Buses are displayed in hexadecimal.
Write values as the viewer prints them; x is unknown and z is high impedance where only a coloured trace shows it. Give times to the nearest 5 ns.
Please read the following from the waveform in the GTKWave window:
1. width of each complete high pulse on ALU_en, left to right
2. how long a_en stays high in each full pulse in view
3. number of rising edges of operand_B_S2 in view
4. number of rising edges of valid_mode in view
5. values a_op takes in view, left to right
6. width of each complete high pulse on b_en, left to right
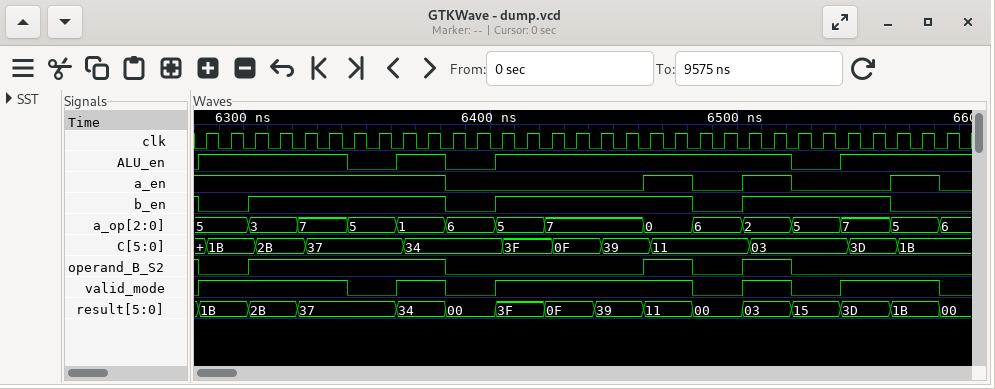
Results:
60 ns, 20 ns, 120 ns
20 ns, 20 ns, 20 ns
3
5
5, 3, 7, 5, 1, 6, 5, 7, 0, 6, 2, 5, 7, 5, 6
80 ns, 80 ns, 60 ns
